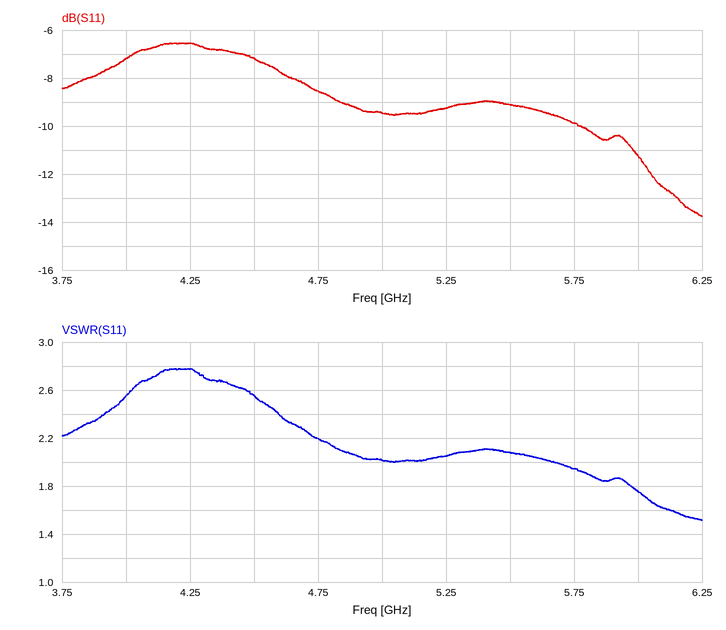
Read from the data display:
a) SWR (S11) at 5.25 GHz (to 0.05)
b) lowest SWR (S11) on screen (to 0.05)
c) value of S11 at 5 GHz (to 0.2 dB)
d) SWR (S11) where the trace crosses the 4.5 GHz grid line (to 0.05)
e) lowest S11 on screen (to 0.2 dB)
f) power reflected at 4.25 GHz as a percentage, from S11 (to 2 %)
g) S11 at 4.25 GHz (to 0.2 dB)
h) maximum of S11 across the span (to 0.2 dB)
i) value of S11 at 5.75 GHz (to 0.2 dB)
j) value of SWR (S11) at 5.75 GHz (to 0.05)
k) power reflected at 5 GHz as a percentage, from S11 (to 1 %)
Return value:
2.05
1.50
-9.4 dB
2.55
-13.8 dB
22 %
-6.6 dB
-6.6 dB
-9.8 dB
1.95
11 %
